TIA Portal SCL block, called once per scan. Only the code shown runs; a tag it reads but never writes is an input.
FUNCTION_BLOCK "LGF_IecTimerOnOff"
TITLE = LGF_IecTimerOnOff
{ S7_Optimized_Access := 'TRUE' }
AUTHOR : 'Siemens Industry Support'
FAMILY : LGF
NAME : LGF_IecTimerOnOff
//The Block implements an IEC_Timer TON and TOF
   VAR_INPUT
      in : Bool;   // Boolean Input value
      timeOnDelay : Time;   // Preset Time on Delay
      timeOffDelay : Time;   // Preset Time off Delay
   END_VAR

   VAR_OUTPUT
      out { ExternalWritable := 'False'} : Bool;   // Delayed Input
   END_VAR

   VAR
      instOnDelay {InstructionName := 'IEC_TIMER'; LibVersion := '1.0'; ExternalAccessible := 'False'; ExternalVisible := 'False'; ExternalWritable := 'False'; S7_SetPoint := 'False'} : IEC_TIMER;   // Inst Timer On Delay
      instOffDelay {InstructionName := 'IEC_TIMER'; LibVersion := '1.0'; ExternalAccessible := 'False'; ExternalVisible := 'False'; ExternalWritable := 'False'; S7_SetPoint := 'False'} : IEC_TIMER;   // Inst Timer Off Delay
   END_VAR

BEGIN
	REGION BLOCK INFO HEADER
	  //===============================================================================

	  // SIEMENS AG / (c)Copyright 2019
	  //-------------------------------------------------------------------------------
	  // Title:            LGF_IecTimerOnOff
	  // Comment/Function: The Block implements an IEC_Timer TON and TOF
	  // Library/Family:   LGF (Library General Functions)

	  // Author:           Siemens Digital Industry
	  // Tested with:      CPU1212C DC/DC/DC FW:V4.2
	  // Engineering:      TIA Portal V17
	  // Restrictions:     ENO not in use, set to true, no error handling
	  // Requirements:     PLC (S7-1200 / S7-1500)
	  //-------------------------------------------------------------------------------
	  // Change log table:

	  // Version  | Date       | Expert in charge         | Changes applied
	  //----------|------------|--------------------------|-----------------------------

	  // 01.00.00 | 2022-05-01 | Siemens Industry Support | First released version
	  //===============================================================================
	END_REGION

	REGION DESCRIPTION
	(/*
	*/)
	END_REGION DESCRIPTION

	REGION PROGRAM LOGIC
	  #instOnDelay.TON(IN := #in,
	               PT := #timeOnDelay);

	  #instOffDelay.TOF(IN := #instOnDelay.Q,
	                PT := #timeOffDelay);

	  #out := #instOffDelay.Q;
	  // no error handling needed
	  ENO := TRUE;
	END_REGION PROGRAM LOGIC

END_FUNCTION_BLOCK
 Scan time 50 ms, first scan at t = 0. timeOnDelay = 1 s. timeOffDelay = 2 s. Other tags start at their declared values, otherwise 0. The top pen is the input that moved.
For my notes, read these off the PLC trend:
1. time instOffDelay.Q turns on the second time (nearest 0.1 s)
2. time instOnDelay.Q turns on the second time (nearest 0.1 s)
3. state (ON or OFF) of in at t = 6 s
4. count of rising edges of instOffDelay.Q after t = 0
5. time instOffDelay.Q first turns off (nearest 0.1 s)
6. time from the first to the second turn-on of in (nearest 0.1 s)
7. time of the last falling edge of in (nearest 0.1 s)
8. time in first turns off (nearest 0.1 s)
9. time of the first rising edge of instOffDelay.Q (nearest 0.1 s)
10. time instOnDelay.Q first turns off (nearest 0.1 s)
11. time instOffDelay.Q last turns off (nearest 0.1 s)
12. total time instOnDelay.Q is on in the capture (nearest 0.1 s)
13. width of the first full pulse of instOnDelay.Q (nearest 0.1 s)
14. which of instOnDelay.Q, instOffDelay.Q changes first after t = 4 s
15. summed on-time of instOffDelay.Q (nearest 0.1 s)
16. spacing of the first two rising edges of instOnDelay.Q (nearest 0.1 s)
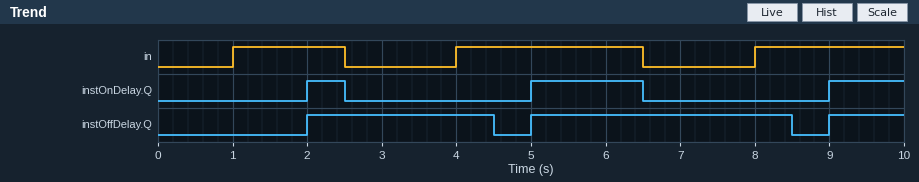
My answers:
5.0 s
5.0 s
ON
3
4.5 s
3.0 s
6.5 s
2.5 s
2.0 s
2.5 s
8.5 s
3.0 s
0.5 s
instOffDelay.Q
7.0 s
3.0 s
